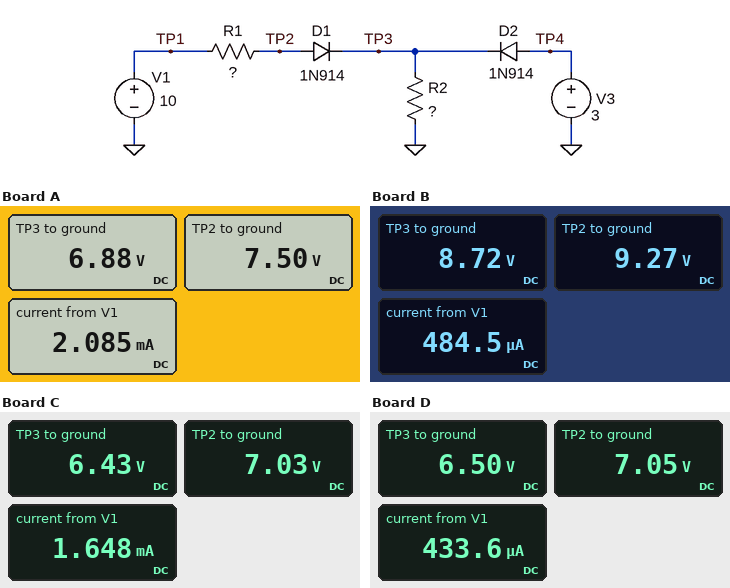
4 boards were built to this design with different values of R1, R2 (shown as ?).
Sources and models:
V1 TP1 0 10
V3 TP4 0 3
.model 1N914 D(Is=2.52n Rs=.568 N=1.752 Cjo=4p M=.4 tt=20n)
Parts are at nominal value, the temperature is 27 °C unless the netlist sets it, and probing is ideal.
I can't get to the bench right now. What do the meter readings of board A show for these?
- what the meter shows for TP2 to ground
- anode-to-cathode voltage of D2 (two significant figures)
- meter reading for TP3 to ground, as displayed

7.50 V
-3.9 V
6.88 V
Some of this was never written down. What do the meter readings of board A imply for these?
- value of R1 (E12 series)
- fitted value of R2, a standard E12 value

1.2 kΩ
3.3 kΩ
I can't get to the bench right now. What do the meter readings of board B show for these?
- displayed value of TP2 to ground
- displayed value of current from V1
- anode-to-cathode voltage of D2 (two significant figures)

9.27 V
484.5 µA
-5.7 V
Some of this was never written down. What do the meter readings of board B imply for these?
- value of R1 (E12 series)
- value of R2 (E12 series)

1.5 kΩ
18 kΩ
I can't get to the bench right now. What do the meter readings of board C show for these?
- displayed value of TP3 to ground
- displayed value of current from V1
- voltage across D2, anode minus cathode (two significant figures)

6.43 V
1.648 mA
-3.4 V
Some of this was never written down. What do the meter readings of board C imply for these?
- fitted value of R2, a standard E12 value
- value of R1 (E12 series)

3.9 kΩ
1.8 kΩ
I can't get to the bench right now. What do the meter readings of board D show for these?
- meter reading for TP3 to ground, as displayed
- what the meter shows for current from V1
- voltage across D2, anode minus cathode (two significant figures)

6.50 V
433.6 µA
-3.5 V
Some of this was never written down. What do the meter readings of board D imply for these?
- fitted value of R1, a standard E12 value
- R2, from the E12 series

6.8 kΩ
15 kΩ
